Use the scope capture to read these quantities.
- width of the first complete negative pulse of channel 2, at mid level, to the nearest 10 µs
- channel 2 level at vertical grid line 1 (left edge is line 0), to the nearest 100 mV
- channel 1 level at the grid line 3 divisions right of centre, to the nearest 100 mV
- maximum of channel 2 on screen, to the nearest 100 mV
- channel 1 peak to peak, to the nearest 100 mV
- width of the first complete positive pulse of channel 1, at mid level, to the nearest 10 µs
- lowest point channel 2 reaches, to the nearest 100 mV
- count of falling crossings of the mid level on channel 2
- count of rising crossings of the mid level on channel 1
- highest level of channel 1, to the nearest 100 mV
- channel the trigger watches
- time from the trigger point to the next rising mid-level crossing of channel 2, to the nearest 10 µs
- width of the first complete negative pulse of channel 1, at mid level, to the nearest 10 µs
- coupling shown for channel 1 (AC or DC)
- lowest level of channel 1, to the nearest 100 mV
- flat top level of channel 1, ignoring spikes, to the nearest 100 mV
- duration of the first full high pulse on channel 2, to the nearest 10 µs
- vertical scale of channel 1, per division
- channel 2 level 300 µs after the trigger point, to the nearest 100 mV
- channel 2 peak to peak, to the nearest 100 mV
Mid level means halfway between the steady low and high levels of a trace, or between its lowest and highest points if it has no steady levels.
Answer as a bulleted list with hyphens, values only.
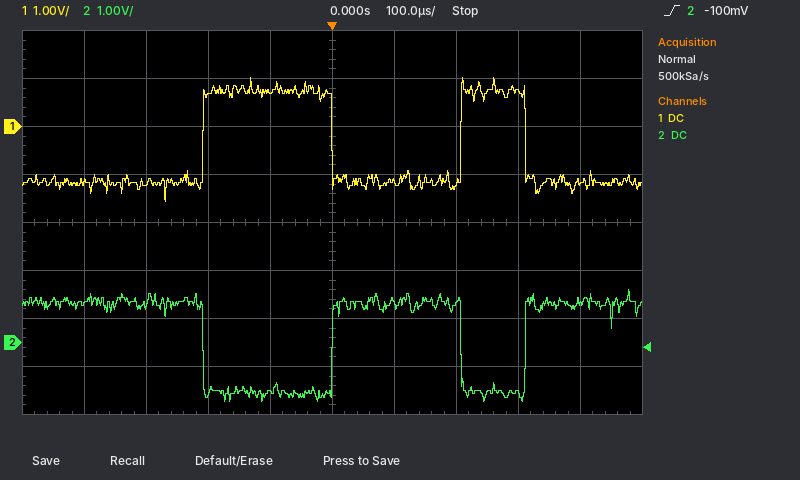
- 210 µs
- 800 mV
- 700 mV
- 1.1 V
- 2.6 V
- 210 µs
- -1.2 V
- 2
- 2
- 1.0 V
- channel 2
- 310 µs
- 210 µs
- DC
- -1.6 V
- 700 mV
- 210 µs
- 1 V
- -1.1 V
- 2.3 V
